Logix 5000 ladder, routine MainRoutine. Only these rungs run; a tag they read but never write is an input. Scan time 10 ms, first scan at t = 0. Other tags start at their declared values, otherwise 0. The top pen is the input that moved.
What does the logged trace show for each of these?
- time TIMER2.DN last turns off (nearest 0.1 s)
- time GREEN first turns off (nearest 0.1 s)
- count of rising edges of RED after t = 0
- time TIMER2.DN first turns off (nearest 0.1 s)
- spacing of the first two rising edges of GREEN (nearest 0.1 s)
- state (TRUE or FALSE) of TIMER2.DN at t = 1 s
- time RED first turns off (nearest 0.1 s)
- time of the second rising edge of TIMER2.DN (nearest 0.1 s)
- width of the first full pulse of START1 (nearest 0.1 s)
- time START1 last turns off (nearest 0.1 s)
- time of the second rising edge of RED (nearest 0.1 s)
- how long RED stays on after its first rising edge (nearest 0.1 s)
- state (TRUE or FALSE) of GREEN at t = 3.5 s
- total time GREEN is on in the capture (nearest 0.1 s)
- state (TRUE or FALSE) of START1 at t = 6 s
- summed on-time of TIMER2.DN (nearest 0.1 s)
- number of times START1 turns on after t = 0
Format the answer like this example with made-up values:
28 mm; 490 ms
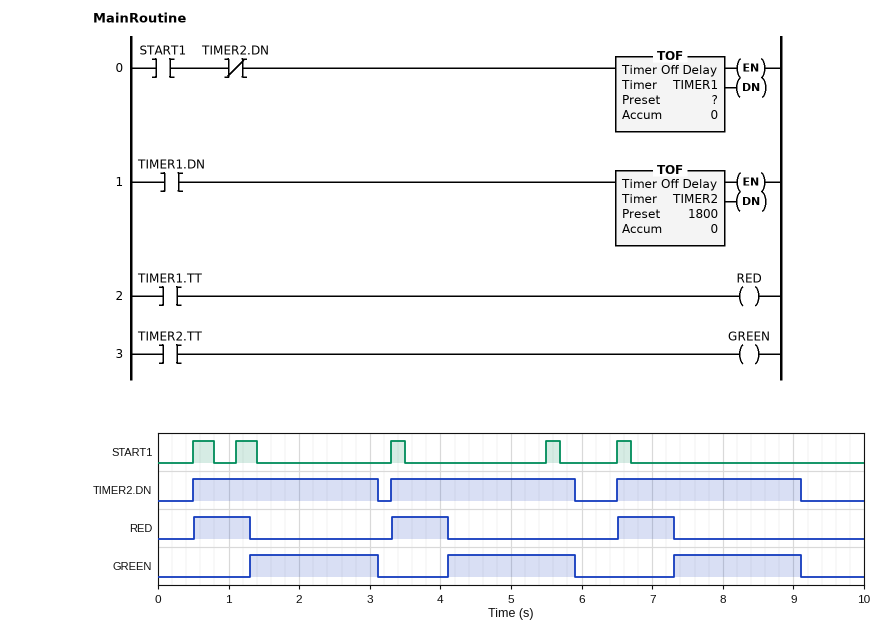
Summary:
9.1 s; 3.1 s; 3; 3.1 s; 2.8 s; TRUE; 1.3 s; 3.3 s; 0.3 s; 6.7 s; 3.3 s; 0.8 s; FALSE; 5.4 s; FALSE; 7.8 s; 5
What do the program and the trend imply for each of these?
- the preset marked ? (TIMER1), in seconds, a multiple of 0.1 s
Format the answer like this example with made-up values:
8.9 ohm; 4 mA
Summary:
0.8 s
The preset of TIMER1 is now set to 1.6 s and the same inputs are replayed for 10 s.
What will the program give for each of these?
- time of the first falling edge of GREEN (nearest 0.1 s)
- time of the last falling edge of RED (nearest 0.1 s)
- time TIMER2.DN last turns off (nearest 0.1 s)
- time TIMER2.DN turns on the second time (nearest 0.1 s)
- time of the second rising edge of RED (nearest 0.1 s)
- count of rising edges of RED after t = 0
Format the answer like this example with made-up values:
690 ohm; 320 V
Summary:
3.9 s; 7.1 s; 8.9 s; 5.5 s; 5.5 s; 2
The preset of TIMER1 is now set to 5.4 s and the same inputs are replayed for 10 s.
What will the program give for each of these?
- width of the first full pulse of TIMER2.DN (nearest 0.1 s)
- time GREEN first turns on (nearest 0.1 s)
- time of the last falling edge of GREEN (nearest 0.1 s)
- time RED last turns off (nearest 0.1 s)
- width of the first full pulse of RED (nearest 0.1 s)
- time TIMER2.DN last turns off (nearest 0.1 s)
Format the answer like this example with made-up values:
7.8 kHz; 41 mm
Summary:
7.2 s; 5.9 s; 7.7 s; 5.9 s; 5.4 s; 7.7 s
